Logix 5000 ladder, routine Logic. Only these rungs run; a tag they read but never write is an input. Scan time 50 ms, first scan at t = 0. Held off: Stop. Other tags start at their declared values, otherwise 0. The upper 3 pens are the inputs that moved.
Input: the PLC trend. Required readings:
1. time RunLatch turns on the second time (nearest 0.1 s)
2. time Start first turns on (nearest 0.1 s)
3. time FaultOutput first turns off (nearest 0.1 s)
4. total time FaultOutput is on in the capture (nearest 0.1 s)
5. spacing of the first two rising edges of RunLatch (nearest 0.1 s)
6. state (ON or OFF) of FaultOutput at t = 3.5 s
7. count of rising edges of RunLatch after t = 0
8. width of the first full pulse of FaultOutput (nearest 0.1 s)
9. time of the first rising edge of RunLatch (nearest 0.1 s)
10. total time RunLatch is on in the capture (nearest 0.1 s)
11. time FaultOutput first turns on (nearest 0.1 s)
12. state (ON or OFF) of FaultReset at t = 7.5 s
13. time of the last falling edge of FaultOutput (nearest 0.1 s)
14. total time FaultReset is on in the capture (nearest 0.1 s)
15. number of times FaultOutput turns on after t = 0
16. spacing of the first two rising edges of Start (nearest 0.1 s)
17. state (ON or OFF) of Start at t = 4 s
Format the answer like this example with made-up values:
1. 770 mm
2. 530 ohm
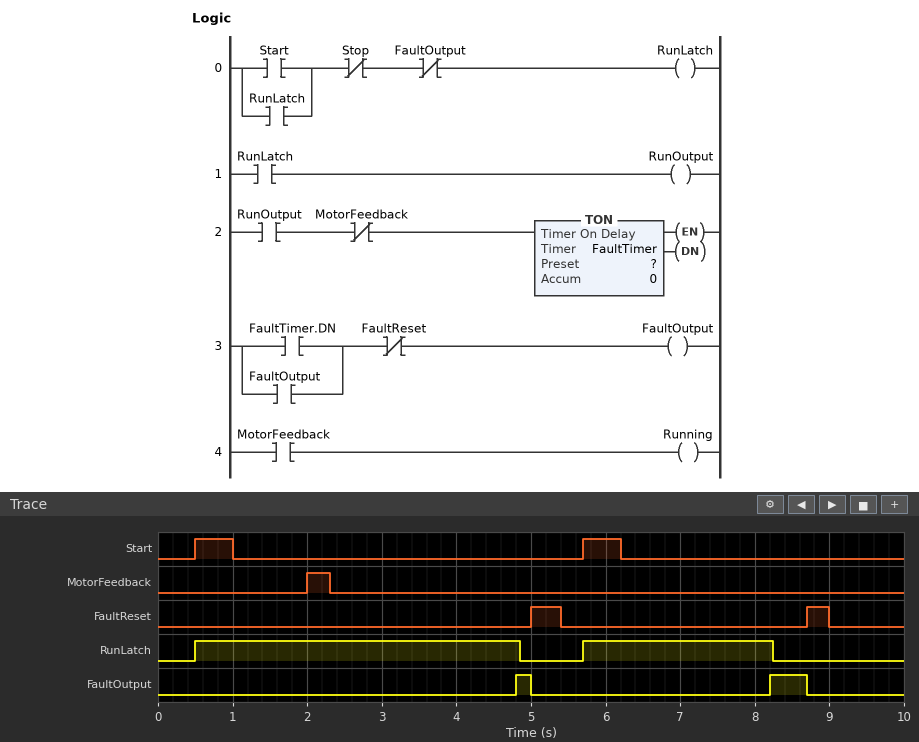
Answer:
1. 5.7 s
2. 0.5 s
3. 5.0 s
4. 0.7 s
5. 5.2 s
6. OFF
7. 2
8. 0.2 s
9. 0.5 s
10. 6.9 s
11. 4.8 s
12. OFF
13. 8.7 s
14. 0.7 s
15. 2
16. 5.2 s
17. OFF
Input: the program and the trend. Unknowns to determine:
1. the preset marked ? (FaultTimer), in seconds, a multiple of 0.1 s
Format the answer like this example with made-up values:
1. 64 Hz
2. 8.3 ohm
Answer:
1. 2.5 s
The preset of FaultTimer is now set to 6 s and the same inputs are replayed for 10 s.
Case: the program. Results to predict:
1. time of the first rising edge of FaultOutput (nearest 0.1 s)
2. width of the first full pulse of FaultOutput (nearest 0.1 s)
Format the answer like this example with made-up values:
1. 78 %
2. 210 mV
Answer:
1. 8.3 s
2. 0.4 s
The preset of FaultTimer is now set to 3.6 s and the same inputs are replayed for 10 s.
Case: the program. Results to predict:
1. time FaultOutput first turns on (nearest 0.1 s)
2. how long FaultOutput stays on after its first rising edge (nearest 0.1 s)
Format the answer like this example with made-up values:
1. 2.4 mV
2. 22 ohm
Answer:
1. 5.9 s
2. 2.8 s
